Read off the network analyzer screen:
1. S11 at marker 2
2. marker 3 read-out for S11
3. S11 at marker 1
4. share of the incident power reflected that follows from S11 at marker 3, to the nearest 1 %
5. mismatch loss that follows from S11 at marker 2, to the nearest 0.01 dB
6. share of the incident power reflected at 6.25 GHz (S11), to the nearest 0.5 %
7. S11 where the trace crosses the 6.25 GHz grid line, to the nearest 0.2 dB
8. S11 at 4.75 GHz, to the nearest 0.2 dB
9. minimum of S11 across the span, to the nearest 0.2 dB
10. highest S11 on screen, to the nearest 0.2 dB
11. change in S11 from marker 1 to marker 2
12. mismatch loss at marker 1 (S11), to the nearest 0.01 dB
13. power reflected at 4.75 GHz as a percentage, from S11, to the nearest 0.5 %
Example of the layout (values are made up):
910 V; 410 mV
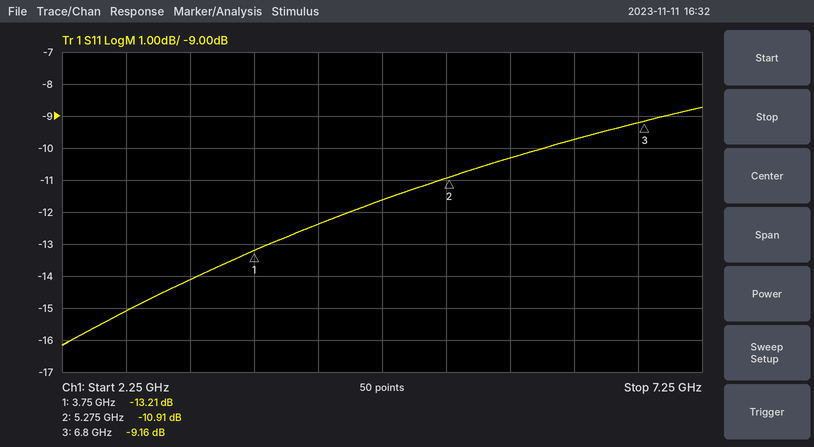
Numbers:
-10.91 dB; -9.16 dB; -13.21 dB; 12 %; 0.37 dB; 10.5 %; -9.8 dB; -11.6 dB; -16.2 dB; -8.8 dB; 2.30 dB; 0.21 dB; 7.0 %
